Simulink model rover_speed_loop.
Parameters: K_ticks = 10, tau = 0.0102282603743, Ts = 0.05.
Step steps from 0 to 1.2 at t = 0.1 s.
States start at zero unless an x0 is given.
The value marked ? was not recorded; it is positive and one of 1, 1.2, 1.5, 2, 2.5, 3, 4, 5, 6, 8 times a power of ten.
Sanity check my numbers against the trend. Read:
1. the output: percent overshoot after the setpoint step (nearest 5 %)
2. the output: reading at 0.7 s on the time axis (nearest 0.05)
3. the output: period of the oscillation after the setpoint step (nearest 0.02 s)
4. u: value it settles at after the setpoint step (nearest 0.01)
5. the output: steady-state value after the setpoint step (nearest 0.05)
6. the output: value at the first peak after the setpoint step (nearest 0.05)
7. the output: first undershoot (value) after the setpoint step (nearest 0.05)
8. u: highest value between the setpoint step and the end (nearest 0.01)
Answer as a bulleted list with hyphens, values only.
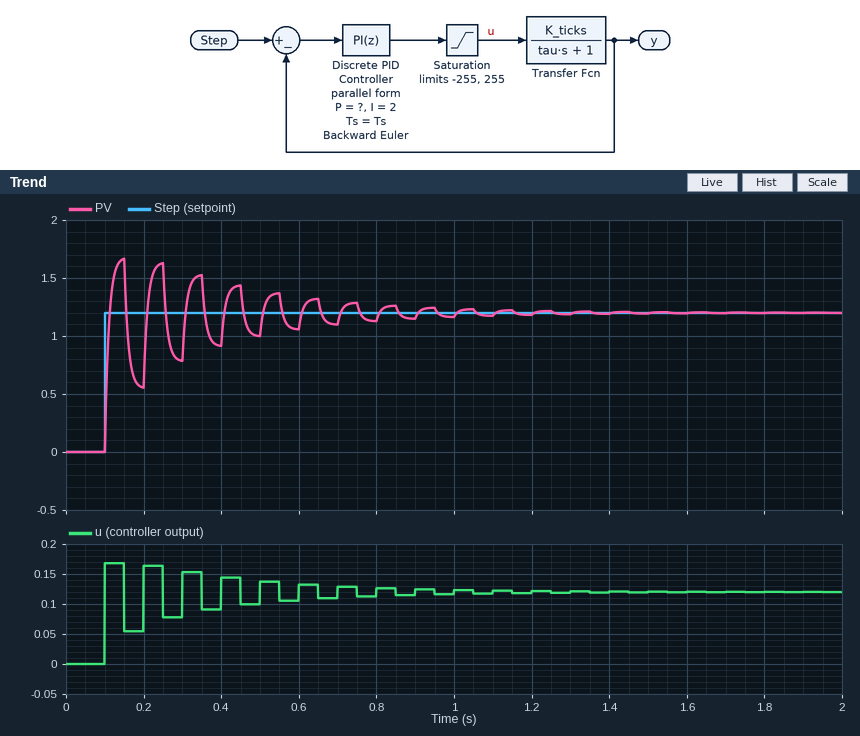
- 40 %
- 1.10
- 0.10 s
- 0.12
- 1.20
- 1.65
- 0.55
- 0.17
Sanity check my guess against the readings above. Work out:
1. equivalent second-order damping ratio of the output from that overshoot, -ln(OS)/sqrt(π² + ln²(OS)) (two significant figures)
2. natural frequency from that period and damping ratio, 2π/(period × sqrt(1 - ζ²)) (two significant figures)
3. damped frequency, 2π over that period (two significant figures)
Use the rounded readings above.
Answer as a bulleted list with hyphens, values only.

- 0.28
- 65 rad/s
- 63 rad/s
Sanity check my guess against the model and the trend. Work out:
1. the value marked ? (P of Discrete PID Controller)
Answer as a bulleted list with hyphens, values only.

- 0.04
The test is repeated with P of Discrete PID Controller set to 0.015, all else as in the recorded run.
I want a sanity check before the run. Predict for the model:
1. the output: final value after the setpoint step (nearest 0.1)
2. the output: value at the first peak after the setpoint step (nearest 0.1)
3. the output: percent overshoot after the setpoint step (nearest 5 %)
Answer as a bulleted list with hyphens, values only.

- 1.2
- 1.4
- 15 %
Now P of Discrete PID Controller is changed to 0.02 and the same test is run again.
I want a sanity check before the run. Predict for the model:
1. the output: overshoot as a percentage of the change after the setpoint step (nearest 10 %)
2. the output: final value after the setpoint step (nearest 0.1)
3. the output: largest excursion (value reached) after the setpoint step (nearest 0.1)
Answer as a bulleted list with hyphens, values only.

- 20 %
- 1.2
- 1.4
